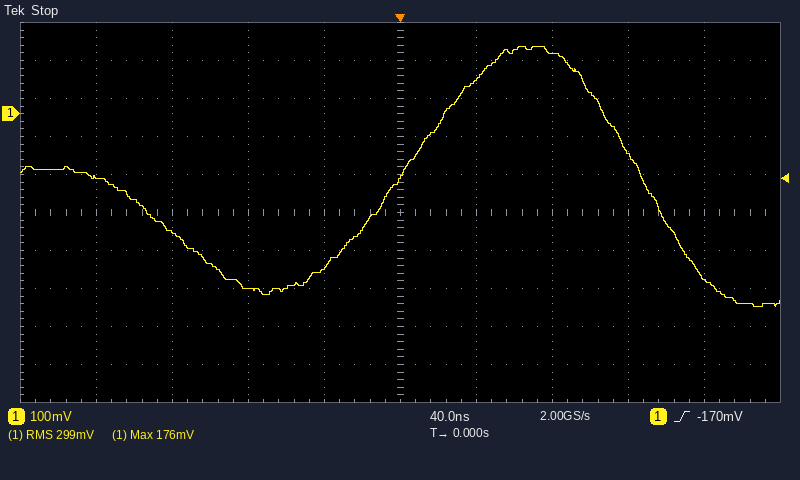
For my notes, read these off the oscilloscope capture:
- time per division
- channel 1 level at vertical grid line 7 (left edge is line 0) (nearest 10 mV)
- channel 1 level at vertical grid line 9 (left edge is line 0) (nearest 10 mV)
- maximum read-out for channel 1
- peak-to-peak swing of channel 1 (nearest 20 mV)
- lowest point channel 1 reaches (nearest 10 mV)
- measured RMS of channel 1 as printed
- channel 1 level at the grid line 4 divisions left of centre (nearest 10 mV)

40 ns
160 mV
-430 mV
176 mV
680 mV
-510 mV
299 mV
-170 mV
